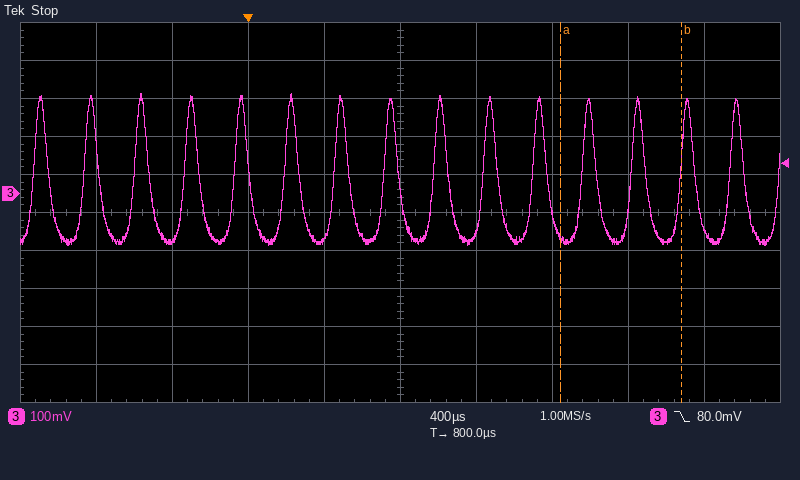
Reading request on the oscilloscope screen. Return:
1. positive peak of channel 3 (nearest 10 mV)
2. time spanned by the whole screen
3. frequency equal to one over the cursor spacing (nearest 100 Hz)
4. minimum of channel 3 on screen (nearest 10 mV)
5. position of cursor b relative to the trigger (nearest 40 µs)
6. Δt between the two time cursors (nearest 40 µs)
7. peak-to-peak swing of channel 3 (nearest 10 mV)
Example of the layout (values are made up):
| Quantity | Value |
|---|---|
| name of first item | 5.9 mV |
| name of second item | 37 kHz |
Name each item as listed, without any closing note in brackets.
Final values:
| Quantity | Value |
|---|---|
| positive peak of channel 3 | 260 mV |
| time spanned by the whole screen | 4 ms |
| frequency equal to one over the cursor spacing | 1.6 kHz |
| minimum of channel 3 on screen | -140 mV |
| position of cursor b relative to the trigger | +2.28 ms |
| Δt between the two time cursors | 640 µs |
| peak-to-peak swing of channel 3 | 400 mV |
